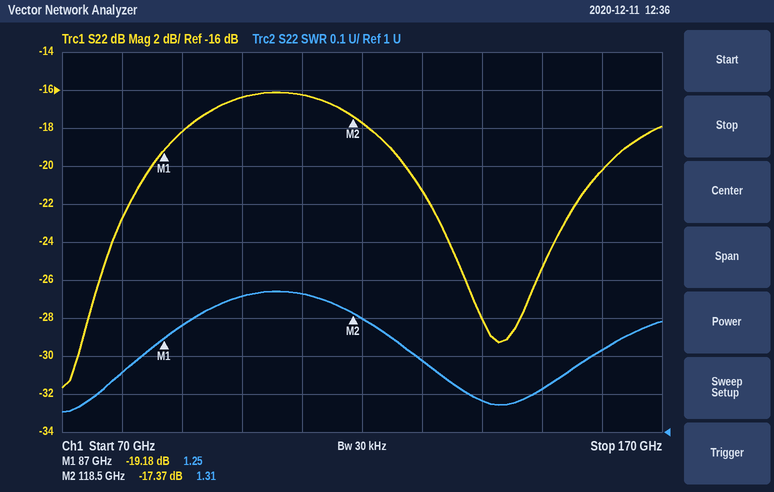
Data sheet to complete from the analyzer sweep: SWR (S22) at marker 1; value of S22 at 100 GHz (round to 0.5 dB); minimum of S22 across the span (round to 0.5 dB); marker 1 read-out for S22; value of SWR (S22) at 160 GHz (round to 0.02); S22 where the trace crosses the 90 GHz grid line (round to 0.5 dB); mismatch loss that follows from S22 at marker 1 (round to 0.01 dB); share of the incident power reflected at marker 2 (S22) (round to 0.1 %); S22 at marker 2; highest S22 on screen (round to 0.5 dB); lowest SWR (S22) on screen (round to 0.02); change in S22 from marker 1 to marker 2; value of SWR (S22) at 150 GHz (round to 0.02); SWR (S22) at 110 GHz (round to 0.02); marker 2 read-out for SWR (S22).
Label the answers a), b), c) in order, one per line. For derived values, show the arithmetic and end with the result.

a) 1.25
b) -16.5 dB
c) -31.5 dB
d) -19.18 dB
e) 1.22
f) -18.0 dB
g) −10 log10(1 − 10^(-19.18/10)) ≈ 0.05 dB
h) 10^(-17.37/10) ≈ 1.8 %
i) -17.37 dB
j) -16.0 dB
k) 1.06
l) -17.37 − (-19.18) = 1.81 dB
m) 1.12
n) 1.36
o) 1.31
